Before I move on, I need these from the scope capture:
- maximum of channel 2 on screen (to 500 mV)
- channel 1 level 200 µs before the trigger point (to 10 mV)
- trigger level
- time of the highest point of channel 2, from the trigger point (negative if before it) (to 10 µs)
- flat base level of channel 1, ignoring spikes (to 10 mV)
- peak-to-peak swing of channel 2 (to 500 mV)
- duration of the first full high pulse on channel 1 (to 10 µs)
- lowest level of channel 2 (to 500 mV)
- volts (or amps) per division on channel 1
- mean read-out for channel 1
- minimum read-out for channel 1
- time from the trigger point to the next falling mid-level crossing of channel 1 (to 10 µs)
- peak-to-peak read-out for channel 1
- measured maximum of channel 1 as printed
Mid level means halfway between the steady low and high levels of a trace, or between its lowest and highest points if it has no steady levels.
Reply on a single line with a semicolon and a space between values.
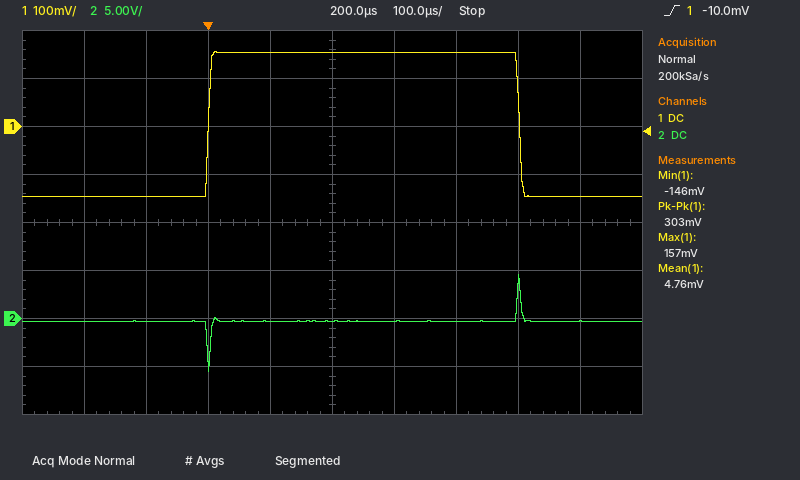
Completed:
4.5 V; -150 mV; -10.0 mV; +500 µs; -150 mV; 10.0 V; 500 µs; -5.5 V; 100 mV; 4.76 mV; -146 mV; 500 µs; 303 mV; 157 mV
